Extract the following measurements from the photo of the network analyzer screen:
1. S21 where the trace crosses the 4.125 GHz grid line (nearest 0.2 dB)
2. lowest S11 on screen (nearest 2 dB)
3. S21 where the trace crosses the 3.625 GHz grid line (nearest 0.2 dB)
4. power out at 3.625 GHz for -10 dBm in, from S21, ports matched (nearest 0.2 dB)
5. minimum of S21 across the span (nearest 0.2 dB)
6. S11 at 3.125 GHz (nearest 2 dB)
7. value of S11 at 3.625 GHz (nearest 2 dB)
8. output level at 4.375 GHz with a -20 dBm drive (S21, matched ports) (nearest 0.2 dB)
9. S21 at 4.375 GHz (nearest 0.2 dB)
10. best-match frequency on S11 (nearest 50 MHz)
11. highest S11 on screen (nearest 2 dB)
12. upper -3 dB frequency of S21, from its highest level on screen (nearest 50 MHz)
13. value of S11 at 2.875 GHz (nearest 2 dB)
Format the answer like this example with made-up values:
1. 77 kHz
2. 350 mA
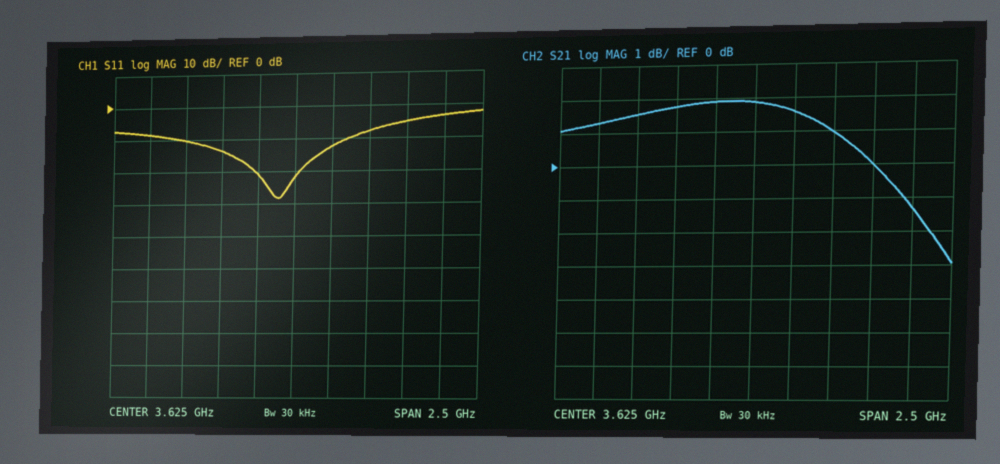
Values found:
1. 1.0 dB
2. -28 dB
3. 1.8 dB
4. -8.2 dBm
5. -3.0 dB
6. -14 dB
7. -22 dB
8. -20.0 dBm
9. 0.0 dB
10. 3.50 GHz
11. -2 dB
12. 4.60 GHz
13. -10 dB
